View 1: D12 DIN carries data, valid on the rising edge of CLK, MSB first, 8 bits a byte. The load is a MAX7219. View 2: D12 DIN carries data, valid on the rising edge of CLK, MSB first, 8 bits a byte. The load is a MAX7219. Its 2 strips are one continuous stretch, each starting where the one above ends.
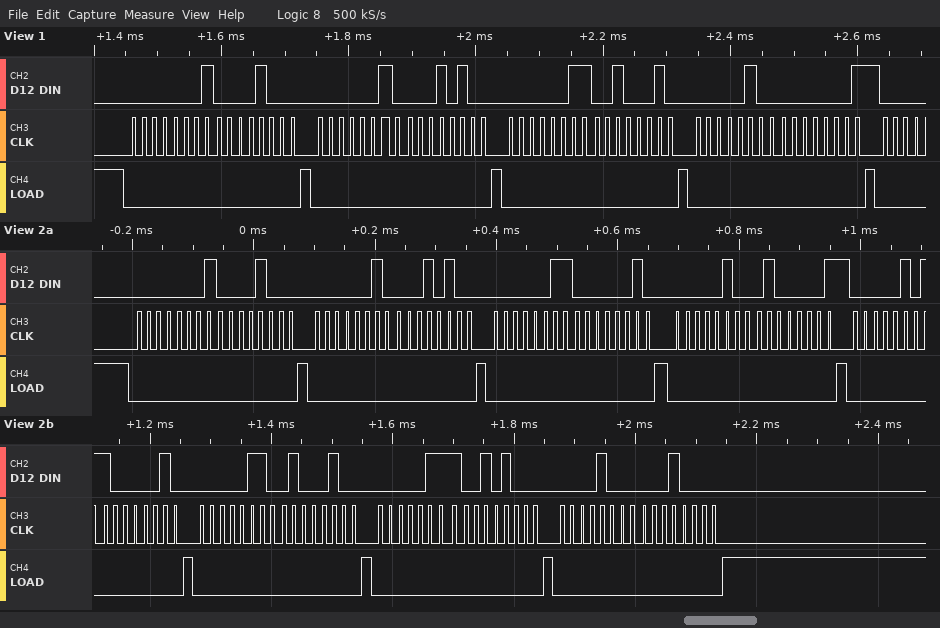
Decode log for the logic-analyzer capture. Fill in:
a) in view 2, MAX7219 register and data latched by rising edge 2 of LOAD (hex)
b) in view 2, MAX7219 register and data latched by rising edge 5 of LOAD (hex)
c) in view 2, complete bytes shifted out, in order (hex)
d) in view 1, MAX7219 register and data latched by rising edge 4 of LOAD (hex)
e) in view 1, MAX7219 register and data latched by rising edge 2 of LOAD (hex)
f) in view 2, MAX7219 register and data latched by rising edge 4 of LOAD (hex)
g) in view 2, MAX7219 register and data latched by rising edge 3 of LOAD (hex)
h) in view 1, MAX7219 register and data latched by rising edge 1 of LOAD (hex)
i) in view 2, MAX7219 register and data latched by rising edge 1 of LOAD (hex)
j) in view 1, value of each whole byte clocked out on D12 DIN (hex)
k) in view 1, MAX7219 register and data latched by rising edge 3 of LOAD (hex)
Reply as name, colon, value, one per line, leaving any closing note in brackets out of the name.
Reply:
in view 2, MAX7219 register and data latched by rising edge 2 of LOAD: register 0x2, data 0x14
in view 2, MAX7219 register and data latched by rising edge 5 of LOAD: register 0x5, data 0x82
in view 2, complete bytes shifted out, in order: 0x01 0x08 0x02 0x14 0x03 0x02 0x04 0x41 0x05 0x82 0x06 0x44 0x07 0x28 0x08 0x10
in view 1, MAX7219 register and data latched by rising edge 4 of LOAD: register 0x4, data 0x01
in view 1, MAX7219 register and data latched by rising edge 2 of LOAD: register 0x2, data 0x14
in view 2, MAX7219 register and data latched by rising edge 4 of LOAD: register 0x4, data 0x41
in view 2, MAX7219 register and data latched by rising edge 3 of LOAD: register 0x3, data 0x02
in view 1, MAX7219 register and data latched by rising edge 1 of LOAD: register 0x1, data 0x08
in view 2, MAX7219 register and data latched by rising edge 1 of LOAD: register 0x1, data 0x08
in view 1, value of each whole byte clocked out on D12 DIN: 01 08 02 14 03 22 04 01
in view 1, MAX7219 register and data latched by rising edge 3 of LOAD: register 0x3, data 0x22
